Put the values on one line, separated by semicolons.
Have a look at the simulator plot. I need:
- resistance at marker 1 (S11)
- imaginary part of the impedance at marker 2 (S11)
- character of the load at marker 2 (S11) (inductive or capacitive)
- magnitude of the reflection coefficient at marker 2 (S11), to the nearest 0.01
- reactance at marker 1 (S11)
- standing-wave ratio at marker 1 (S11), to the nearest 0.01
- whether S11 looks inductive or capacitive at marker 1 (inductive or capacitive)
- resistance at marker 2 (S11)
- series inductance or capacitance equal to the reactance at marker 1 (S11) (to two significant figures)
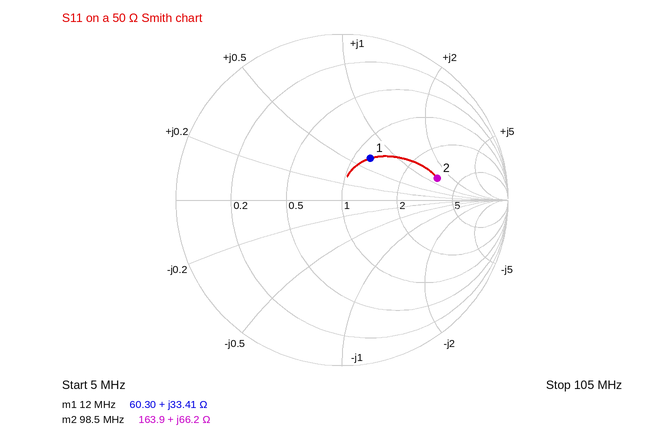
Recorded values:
60.30 Ω; +66.2 Ω; inductive; 0.59; +33.41 Ω; 1.87; inductive; 163.9 Ω; 440 nH
